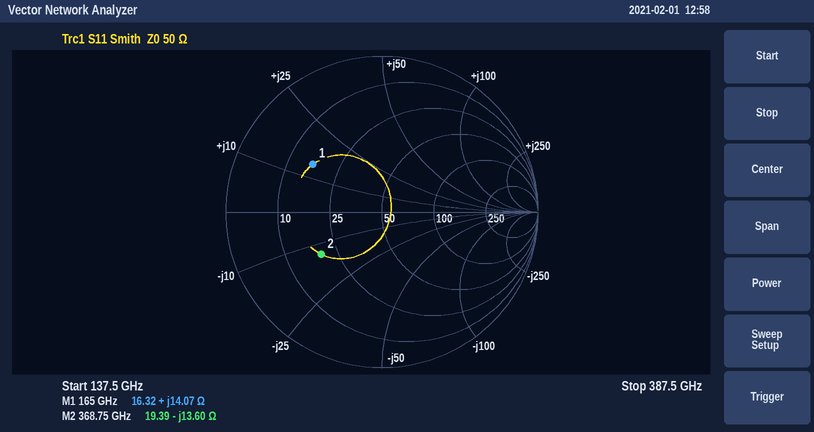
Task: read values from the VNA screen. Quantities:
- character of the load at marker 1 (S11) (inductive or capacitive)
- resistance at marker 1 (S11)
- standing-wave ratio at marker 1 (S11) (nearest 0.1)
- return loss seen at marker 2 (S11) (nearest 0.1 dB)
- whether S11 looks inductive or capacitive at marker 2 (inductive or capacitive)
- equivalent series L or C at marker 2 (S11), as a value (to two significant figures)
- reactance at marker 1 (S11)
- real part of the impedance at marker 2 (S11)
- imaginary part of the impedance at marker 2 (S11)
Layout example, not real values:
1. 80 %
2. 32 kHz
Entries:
1. inductive
2. 16.32 Ω
3. 3.3
4. 6.5 dB
5. capacitive
6. 32 fF
7. +14.07 Ω
8. 19.39 Ω
9. -13.60 Ω
